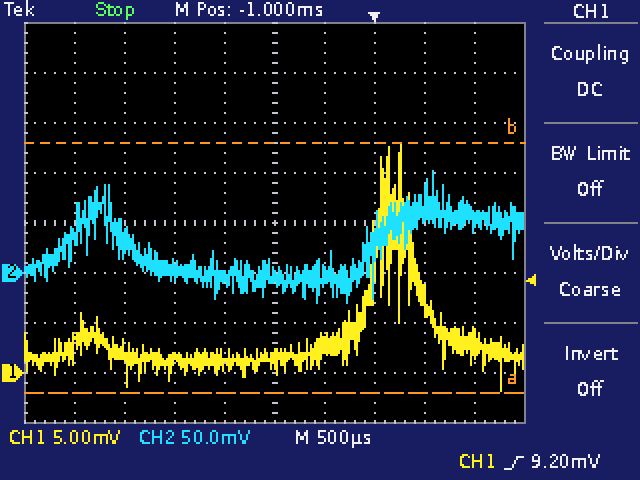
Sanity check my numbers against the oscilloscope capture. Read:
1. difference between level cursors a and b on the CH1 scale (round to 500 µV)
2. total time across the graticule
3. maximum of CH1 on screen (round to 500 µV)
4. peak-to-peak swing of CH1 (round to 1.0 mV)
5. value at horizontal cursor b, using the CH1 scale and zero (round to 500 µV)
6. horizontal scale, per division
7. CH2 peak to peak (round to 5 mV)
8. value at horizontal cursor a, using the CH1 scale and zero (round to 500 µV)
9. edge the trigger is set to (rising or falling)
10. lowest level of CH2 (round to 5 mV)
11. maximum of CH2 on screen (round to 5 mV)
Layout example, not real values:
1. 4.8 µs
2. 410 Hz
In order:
1. 25.0 mV
2. 5 ms
3. 23.0 mV
4. 25.0 mV
5. 23.0 mV
6. 500 µs
7. 130 mV
8. -2.0 mV
9. rising
10. -30 mV
11. 100 mV
